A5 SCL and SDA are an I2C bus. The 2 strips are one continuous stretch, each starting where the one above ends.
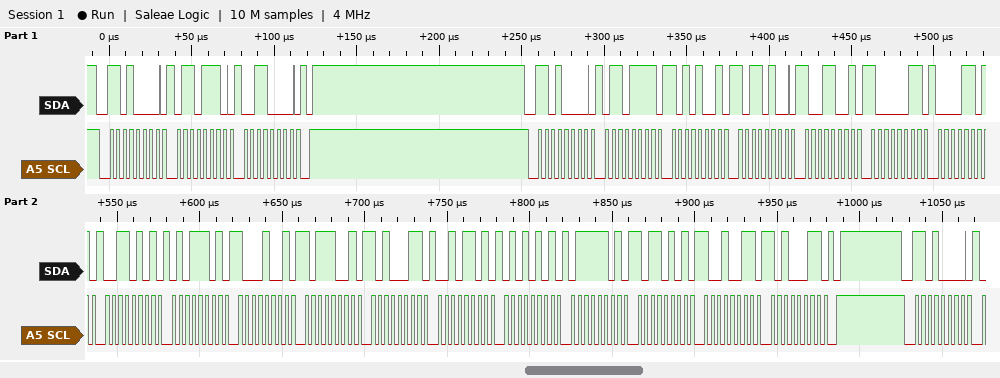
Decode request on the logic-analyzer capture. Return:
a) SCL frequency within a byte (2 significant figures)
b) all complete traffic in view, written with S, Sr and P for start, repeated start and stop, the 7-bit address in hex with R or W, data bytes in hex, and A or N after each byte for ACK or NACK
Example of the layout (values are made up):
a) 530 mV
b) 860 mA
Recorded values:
a) 250 kHz
b) S 68W A 6E A 30 A P S 68W A 6F A A9 A B4 A 99 A 83 A 0D A 35 A 5D A 89 A B9 A A3 A 2D A 55 A 7D A B5 A 93 A A3 A P S 68W A
